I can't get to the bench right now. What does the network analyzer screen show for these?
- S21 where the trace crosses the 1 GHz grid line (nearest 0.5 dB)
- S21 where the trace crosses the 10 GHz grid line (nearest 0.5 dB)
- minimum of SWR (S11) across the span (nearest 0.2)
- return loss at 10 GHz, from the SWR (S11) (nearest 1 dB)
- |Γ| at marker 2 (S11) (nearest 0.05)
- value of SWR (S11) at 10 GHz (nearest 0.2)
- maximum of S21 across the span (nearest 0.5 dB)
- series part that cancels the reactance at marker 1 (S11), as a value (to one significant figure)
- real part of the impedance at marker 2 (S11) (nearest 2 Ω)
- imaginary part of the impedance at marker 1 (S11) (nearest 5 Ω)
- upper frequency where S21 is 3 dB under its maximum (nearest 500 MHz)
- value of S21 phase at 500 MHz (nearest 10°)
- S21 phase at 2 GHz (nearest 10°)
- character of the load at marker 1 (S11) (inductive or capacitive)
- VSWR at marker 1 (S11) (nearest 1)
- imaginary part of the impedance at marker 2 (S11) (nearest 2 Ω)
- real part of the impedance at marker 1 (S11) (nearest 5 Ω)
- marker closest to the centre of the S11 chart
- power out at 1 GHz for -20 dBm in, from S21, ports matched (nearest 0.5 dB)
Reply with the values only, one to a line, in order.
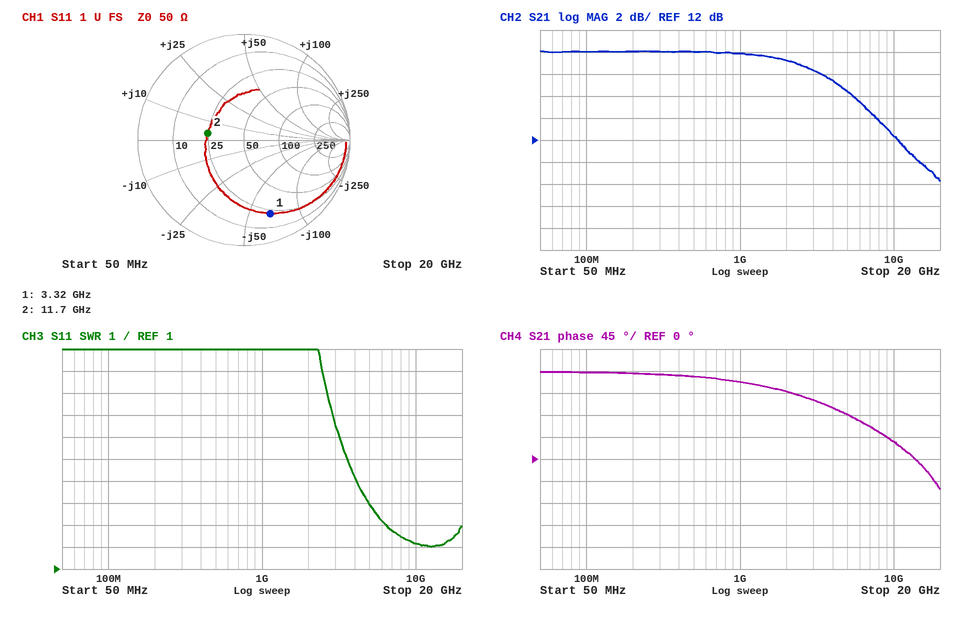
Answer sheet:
20.0 dB
12.5 dB
2.0
9 dB
0.35
2.2
20.0 dB
3 nH
24 Ω
-65 Ω
4.5 GHz
170°
140°
capacitive
7
+4 Ω
20 Ω
marker 2
0.0 dBm
